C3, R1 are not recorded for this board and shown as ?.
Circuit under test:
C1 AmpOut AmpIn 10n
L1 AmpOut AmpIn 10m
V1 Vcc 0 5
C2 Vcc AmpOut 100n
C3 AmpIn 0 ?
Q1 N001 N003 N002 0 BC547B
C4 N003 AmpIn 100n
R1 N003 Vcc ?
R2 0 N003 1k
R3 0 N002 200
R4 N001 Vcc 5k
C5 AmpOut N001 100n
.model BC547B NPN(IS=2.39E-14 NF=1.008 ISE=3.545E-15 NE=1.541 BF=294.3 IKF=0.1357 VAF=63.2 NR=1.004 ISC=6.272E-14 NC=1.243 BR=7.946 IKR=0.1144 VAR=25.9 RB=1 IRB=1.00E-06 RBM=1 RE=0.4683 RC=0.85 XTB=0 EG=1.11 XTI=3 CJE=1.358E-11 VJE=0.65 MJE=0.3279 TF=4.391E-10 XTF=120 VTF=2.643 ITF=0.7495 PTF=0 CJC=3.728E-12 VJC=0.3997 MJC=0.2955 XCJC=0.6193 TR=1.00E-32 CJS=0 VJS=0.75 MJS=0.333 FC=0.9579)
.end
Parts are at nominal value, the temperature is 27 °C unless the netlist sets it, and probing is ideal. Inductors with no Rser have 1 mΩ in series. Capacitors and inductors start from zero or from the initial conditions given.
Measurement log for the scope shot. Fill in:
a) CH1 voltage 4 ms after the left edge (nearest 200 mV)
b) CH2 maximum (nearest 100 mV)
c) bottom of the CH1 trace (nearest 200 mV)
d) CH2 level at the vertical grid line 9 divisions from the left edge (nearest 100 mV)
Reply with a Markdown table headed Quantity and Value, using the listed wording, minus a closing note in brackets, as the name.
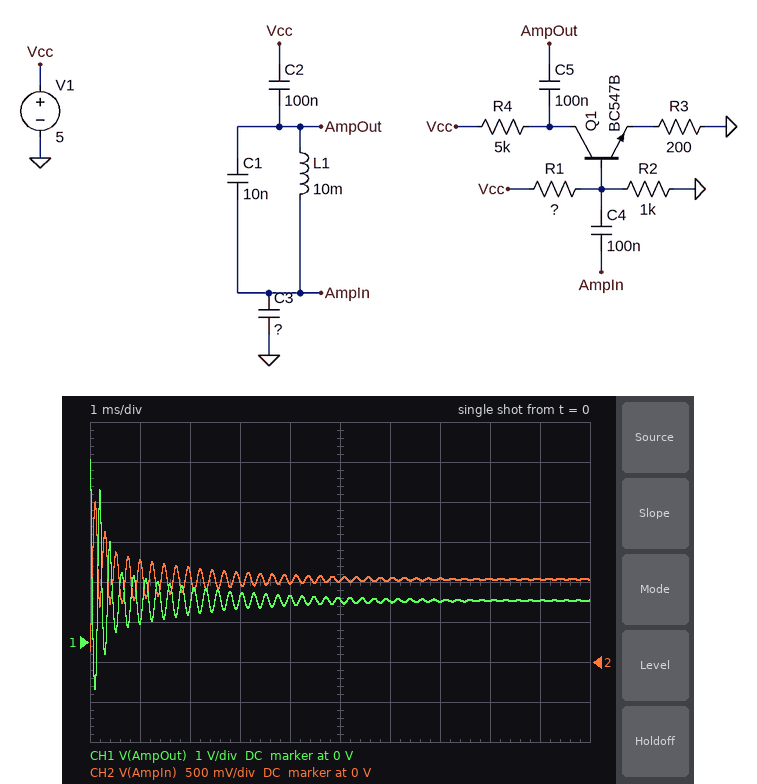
| Quantity | Value |
|---|---|
| CH1 voltage 4 ms after the left edge | 1.2 V |
| CH2 maximum | 2.0 V |
| bottom of the CH1 trace | -1.2 V |
| CH2 level at the vertical grid line 9 divisions from the left edge | 1.0 V |
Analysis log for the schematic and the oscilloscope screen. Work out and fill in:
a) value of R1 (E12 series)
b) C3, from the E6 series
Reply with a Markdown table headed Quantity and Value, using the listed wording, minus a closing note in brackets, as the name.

| Quantity | Value |
|---|---|
| value of R1 | 1.8 kΩ |
| C3, from the E6 series | 330 nF |
